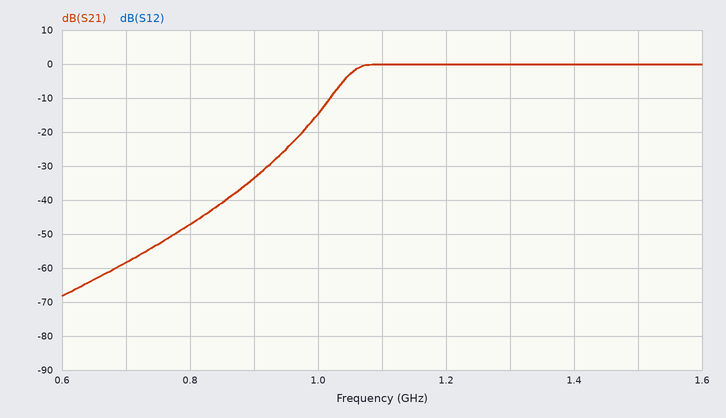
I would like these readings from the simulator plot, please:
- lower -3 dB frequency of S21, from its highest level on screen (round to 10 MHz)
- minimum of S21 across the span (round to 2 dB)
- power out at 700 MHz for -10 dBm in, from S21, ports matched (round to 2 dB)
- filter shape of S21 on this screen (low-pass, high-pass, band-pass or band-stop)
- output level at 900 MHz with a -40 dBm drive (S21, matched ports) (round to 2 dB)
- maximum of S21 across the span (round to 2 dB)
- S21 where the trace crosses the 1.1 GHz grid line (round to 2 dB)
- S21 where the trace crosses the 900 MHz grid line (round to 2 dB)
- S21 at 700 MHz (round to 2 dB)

1.05 GHz
-68 dB
-68 dBm
high-pass
-74 dBm
0 dB
0 dB
-34 dB
-58 dB
